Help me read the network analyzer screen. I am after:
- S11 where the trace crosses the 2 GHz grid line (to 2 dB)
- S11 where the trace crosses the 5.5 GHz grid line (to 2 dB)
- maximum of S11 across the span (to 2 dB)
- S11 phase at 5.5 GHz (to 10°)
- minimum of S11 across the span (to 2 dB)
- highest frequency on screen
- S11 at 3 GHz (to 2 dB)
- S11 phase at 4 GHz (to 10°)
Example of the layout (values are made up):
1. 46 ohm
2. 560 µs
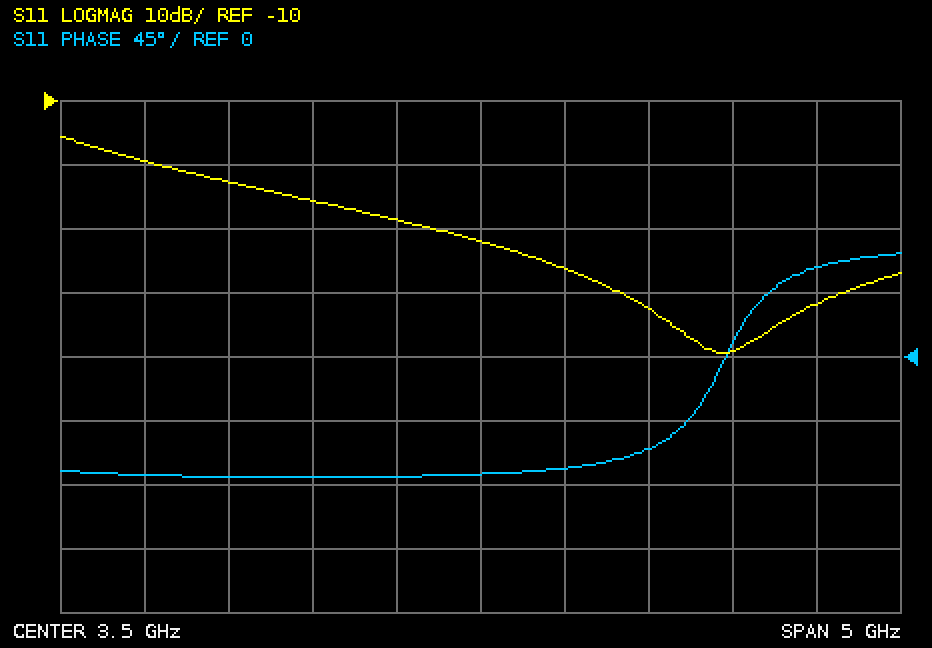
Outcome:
1. -22 dB
2. -42 dB
3. -16 dB
4. 60°
5. -50 dB
6. 6 GHz
7. -28 dB
8. -80°
